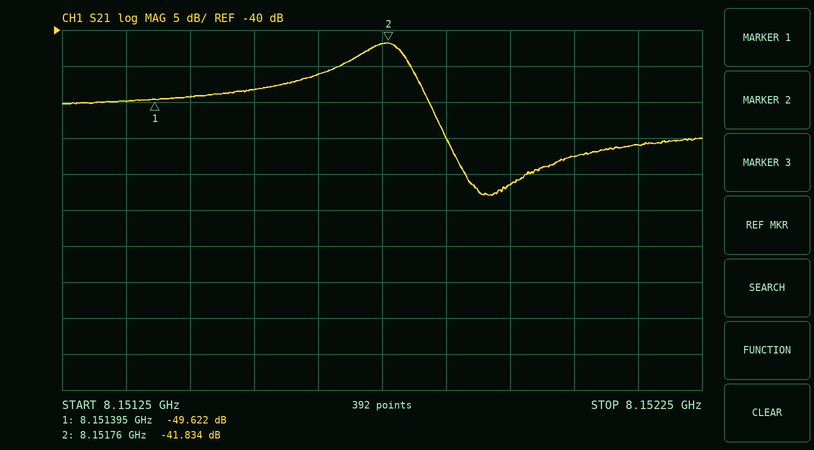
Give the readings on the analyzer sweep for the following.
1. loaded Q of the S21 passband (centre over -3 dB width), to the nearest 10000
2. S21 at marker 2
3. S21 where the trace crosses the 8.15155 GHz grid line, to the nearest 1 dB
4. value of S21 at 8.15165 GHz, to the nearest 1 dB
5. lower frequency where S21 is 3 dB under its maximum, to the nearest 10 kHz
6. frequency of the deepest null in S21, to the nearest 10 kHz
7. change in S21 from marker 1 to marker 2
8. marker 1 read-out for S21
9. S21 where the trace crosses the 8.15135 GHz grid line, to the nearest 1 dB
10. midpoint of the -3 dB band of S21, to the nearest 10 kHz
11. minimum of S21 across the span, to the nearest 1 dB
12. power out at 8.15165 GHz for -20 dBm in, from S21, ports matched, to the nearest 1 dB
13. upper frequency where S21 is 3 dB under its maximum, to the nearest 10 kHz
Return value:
80000
-41.834 dB
-48 dB
-46 dB
8.15169 GHz
8.15192 GHz
7.788 dB
-49.622 dB
-50 dB
8.15174 GHz
-63 dB
-66 dBm
8.15179 GHz
